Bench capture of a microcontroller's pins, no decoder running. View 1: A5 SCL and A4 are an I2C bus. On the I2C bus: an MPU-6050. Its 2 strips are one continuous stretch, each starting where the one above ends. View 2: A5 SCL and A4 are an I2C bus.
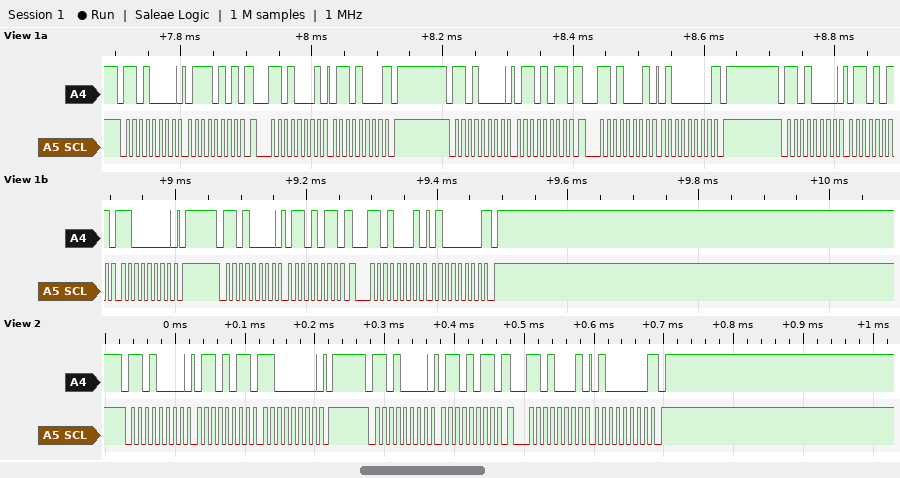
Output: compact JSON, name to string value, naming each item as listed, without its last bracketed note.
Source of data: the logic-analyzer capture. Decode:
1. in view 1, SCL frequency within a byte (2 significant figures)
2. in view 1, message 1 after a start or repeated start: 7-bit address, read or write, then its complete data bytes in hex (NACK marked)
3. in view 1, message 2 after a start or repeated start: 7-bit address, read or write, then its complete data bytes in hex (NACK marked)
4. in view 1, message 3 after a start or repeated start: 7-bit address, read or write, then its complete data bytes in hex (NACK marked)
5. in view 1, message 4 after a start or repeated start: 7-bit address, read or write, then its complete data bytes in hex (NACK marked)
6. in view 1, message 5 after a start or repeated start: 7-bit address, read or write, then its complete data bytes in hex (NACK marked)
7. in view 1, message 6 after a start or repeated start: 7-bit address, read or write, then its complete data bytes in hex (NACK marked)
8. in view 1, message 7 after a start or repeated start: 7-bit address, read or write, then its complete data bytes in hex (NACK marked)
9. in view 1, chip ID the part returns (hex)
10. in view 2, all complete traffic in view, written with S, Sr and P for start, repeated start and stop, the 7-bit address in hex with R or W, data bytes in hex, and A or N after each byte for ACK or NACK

{"in view 1, SCL frequency within a byte": "100 kHz", "in view 1, message 1 after a start or repeated start: 7-bit address, read or write, then its complete data bytes in hex": "0x68 write: 75", "in view 1, message 2 after a start or repeated start: 7-bit address, read or write, then its complete data bytes in hex": "0x68 read: 68 NACK", "in view 1, message 3 after a start or repeated start: 7-bit address, read or write, then its complete data bytes in hex": "0x68 write: 6B", "in view 1, message 4 after a start or repeated start: 7-bit address, read or write, then its complete data bytes in hex": "0x68 read: 40 NACK", "in view 1, message 5 after a start or repeated start: 7-bit address, read or write, then its complete data bytes in hex": "0x68 write: 6B C0", "in view 1, message 6 after a start or repeated start: 7-bit address, read or write, then its complete data bytes in hex": "0x68 write: 6B", "in view 1, message 7 after a start or repeated start: 7-bit address, read or write, then its complete data bytes in hex": "0x68 read: 40 NACK", "in view 1, chip ID the part returns": "0x68", "in view 2, all complete traffic in view, written with S, Sr and P for start, repeated start and stop, the 7-bit address in hex with R or W, data bytes in hex, and A or N after each byte for ACK or NACK": "S 68W A 6B A C0 A P S 68W A 6B A Sr 68R A 40 N P"}
